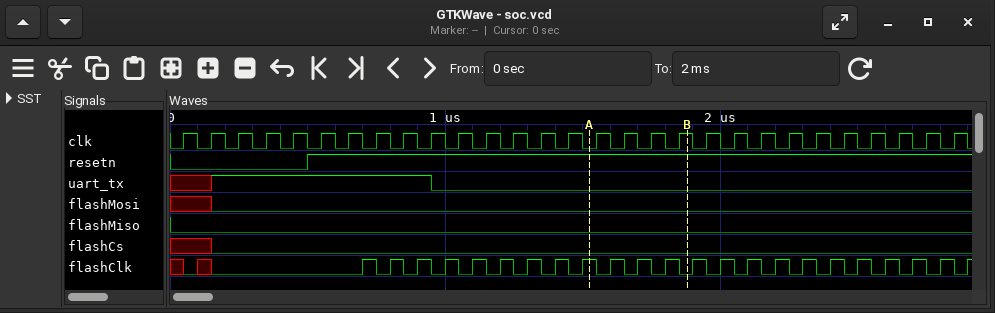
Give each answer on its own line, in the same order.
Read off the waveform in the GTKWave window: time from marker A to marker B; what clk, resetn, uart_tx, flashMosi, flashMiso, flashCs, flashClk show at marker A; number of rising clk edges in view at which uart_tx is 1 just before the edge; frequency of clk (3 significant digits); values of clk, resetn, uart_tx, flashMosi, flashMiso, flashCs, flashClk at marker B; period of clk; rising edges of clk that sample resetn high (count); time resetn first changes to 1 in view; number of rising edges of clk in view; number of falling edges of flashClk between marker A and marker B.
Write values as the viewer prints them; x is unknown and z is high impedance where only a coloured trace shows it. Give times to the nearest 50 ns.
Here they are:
350 ns
clk=0, resetn=1, uart_tx=0, flashMosi=0, flashMiso=0, flashCs=0, flashClk=1
8
10.0 MHz
clk=1, resetn=1, uart_tx=0, flashMosi=0, flashMiso=0, flashCs=0, flashClk=0
100 ns
24
500 ns
29
4
